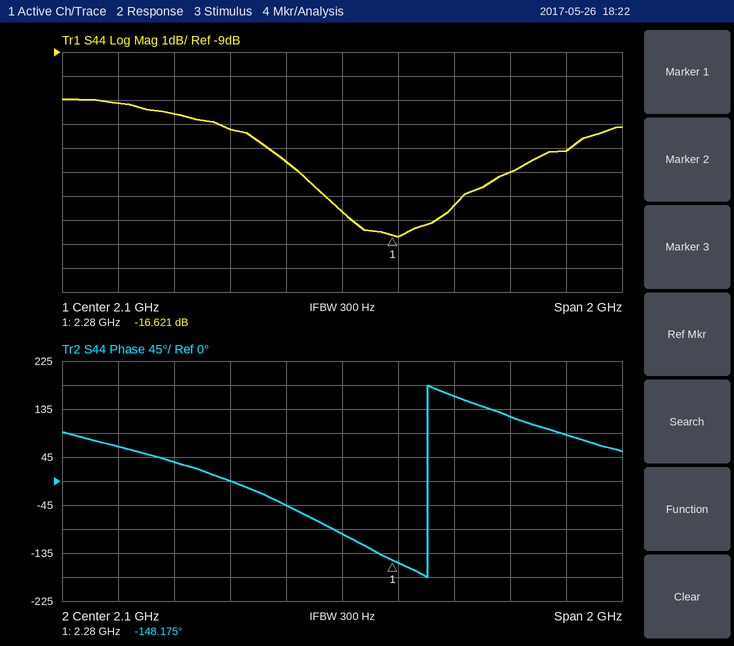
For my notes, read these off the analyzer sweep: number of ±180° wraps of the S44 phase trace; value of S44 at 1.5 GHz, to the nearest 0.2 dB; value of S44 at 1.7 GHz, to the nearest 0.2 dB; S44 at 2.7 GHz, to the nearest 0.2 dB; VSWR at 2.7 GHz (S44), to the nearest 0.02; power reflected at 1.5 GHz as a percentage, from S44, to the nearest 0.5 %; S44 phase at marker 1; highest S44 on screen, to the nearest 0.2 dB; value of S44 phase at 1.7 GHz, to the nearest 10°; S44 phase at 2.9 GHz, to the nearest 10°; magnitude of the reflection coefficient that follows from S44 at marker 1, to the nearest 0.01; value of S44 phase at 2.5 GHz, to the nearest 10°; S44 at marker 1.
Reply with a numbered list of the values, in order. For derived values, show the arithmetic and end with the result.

1. 1
2. -11.6 dB
3. -12.2 dB
4. -14.0 dB
5. |Γ| = 10^(-14/20) = 0.1995; VSWR = (1 + 0.1995)/(1 − 0.1995) ≈ 1.50
6. 10^(-11.6/10) ≈ 6.92 %, so 7.0 % to the nearest 0.5 %
7. -148.175°
8. -11.0 dB
9. 0°
10. 90°
11. 10^(-16.621/20) ≈ 0.15
12. 160°
13. -16.621 dB
